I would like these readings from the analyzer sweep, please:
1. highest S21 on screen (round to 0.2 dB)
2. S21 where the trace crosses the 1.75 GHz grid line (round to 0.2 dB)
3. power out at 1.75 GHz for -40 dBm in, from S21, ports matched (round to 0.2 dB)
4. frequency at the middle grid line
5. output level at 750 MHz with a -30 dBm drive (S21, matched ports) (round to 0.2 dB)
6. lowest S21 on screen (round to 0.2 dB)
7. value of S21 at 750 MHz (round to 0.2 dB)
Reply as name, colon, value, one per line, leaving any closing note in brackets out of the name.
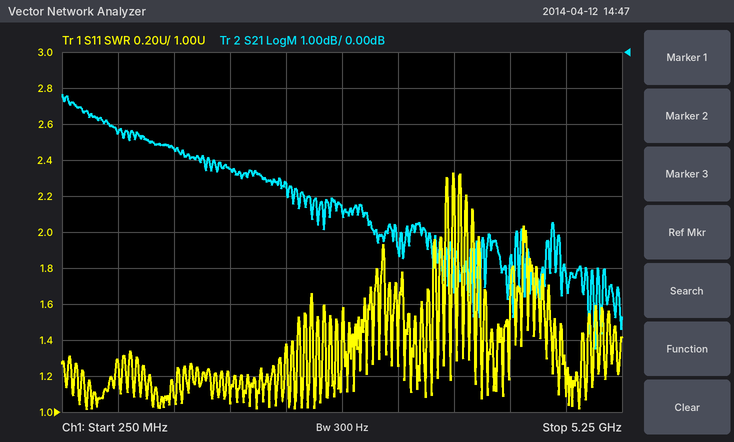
highest S21 on screen: -1.2 dB
S21 where the trace crosses the 1.75 GHz grid line: -3.2 dB
power out at 1.75 GHz for -40 dBm in, from S21, ports matched: -43.2 dBm
frequency at the middle grid line: 2.75 GHz
output level at 750 MHz with a -30 dBm drive (S21, matched ports): -32.2 dBm
lowest S21 on screen: -8.2 dB
value of S21 at 750 MHz: -2.2 dB
